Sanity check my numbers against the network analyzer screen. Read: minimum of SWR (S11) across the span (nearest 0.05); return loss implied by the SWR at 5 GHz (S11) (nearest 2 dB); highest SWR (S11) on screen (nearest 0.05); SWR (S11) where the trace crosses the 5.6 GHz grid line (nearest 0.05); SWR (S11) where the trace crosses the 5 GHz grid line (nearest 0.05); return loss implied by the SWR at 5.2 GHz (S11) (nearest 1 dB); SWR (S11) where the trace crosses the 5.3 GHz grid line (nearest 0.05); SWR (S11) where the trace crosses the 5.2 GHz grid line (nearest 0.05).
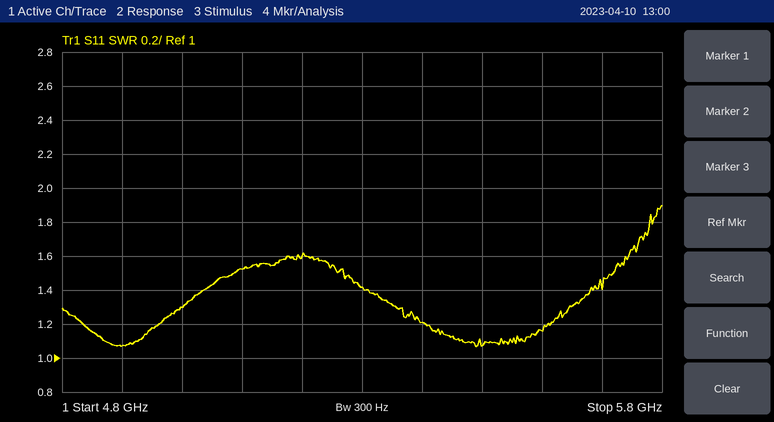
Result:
1.05
18 dB
1.90
1.15
1.30
13 dB
1.40
1.60
